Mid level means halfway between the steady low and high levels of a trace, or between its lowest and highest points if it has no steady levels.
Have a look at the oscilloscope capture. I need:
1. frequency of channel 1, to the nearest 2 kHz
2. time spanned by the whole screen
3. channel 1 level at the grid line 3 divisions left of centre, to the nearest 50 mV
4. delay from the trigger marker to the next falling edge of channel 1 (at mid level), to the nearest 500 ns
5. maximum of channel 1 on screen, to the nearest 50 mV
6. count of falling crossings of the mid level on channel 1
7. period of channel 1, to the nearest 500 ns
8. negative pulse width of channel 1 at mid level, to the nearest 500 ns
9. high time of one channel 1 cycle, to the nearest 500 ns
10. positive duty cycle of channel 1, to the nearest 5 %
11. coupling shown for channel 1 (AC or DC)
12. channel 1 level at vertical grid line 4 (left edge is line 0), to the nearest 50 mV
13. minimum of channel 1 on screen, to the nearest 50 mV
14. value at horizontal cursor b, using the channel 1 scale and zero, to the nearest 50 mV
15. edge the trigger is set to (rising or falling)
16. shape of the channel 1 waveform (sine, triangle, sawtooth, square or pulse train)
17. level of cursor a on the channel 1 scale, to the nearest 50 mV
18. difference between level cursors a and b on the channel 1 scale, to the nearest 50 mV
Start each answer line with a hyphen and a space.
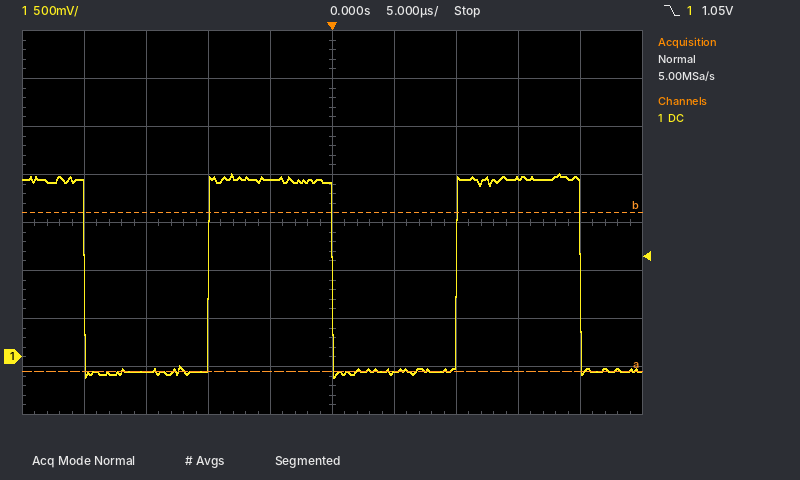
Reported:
- 50 kHz
- 50 µs
- -150 mV
- 20.0 µs
- 1.90 V
- 3
- 20.0 µs
- 10.0 µs
- 10.0 µs
- 50 %
- DC
- 1.85 V
- -200 mV
- 1.50 V
- falling
- square
- -150 mV
- 1.65 V
